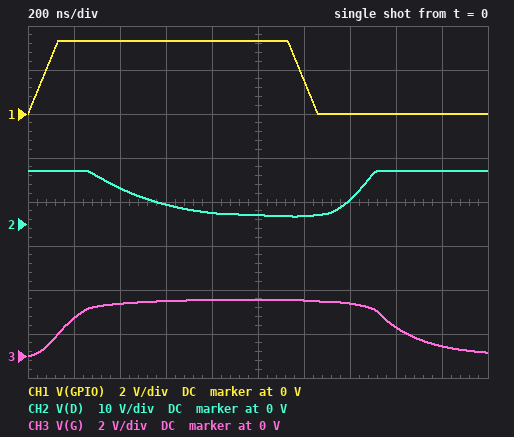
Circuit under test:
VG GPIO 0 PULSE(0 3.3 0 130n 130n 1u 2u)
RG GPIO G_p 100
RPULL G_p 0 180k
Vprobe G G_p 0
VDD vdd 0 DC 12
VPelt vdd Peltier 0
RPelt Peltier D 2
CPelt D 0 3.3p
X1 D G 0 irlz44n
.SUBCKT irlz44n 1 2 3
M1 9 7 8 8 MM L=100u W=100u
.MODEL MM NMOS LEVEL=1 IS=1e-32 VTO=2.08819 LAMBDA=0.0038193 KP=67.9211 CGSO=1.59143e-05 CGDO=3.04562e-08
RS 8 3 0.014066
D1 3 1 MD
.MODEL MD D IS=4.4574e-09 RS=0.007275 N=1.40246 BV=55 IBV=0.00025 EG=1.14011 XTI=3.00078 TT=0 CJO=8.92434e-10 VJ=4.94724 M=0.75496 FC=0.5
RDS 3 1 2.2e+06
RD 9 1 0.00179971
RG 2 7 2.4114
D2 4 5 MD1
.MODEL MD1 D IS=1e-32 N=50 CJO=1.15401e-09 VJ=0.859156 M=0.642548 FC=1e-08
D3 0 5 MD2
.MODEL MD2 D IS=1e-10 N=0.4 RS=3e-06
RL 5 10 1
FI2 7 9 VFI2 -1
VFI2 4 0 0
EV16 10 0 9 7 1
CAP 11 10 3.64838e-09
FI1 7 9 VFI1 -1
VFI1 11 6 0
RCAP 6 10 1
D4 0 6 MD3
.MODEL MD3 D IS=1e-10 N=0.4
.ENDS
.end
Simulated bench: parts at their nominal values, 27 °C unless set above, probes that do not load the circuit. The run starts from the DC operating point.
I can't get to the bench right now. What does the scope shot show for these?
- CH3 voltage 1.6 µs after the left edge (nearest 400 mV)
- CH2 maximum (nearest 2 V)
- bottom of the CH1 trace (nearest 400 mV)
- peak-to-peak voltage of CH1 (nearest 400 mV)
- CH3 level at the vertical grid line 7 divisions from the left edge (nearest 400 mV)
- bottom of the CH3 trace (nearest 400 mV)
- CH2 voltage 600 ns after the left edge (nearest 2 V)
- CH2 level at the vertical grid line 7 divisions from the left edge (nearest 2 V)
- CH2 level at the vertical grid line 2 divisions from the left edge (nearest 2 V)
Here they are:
1.2 V
12 V
0 V
3.2 V
2.4 V
0 V
4 V
6 V
8 V
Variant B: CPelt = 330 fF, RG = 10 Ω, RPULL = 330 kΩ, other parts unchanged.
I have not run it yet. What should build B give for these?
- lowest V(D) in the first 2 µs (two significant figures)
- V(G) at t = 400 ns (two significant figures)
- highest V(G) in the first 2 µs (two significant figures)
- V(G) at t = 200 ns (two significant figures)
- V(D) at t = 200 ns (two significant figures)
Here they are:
170 mV
3.1 V
3.3 V
2.7 V
2.0 V
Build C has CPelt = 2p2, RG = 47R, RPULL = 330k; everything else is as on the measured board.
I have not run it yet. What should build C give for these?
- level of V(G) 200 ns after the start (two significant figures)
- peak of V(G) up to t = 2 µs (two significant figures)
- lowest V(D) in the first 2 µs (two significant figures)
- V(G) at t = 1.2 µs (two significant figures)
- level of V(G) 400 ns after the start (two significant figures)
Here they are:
2.3 V
2.9 V
220 mV
2.7 V
2.6 V
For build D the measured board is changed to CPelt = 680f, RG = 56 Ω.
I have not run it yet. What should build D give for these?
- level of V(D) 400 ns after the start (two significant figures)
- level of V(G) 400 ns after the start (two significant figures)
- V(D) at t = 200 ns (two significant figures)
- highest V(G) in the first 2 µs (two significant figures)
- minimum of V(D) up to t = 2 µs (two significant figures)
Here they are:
3.8 V
2.5 V
11 V
2.7 V
310 mV
